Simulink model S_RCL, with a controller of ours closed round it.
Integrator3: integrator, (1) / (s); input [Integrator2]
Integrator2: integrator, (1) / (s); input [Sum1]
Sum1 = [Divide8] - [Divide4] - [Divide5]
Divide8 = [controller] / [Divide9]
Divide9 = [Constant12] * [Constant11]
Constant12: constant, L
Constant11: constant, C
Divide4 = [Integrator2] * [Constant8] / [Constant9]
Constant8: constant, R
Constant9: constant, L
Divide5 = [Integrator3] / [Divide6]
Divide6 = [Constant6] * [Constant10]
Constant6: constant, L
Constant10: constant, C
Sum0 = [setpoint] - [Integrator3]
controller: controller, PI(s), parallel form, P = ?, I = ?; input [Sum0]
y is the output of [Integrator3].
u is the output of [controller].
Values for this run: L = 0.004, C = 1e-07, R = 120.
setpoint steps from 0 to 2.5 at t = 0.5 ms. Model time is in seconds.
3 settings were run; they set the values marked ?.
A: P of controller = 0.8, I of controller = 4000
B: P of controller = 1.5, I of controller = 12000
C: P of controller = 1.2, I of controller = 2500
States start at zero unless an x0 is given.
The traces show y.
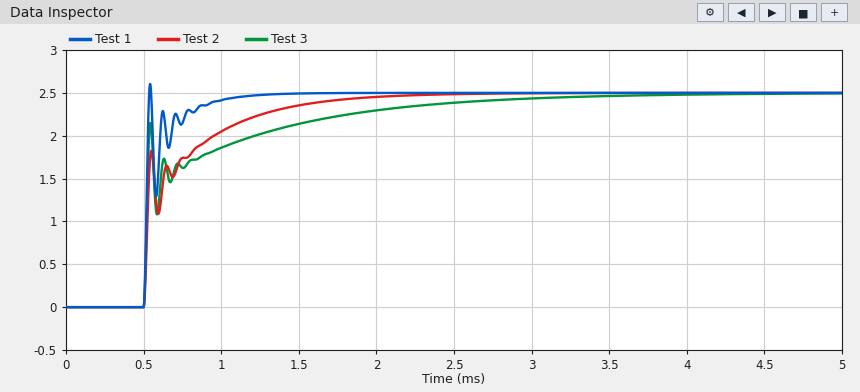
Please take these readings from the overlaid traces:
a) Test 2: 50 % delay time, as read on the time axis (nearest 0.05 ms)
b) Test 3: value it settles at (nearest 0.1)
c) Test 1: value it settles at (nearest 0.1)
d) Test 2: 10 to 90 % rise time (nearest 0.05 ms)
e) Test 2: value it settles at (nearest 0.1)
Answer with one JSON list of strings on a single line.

["0.55 ms", "2.5", "2.5", "0.75 ms", "2.5"]
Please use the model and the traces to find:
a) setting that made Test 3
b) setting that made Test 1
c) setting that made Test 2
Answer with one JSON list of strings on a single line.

["C", "B", "A"]
